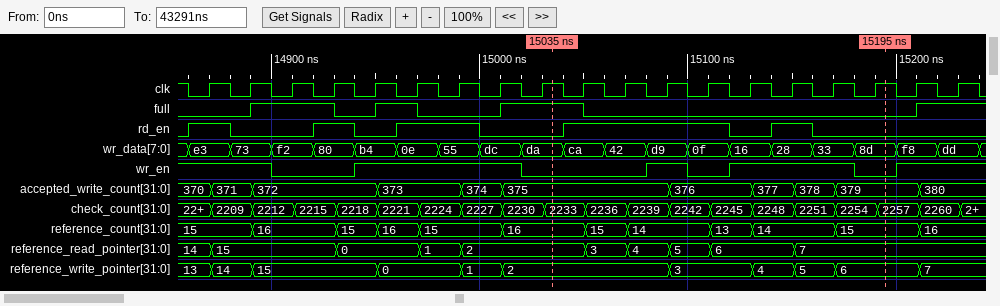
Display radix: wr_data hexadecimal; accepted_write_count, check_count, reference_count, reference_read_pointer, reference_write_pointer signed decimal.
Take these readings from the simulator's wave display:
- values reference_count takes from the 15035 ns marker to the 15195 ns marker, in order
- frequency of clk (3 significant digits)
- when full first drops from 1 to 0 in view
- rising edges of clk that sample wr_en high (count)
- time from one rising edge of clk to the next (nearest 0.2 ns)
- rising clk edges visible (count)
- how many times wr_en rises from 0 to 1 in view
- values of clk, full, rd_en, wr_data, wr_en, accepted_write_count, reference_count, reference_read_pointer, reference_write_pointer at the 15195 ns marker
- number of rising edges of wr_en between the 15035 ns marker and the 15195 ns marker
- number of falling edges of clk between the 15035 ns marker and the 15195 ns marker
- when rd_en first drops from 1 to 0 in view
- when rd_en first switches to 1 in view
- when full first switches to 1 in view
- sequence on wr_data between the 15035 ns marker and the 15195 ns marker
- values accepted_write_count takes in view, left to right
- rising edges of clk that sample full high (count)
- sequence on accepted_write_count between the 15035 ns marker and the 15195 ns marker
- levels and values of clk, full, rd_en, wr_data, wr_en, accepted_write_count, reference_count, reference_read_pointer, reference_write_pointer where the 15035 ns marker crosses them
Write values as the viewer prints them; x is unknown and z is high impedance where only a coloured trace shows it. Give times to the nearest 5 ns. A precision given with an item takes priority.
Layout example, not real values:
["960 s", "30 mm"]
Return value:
["16, 15, 14, 13, 14, 15", "50.0 MHz", "14930 ns", "12", "20 ns", "19", "4", "clk=1, full=0, rd_en=0, wr_data=8d, wr_en=0, accepted_write_count=379, reference_count=15, reference_read_pointer=7, reference_write_pointer=6", "2", "8", "14880 ns", "14860 ns", "14890 ns", "da, ca, 42, d9, 0f, 16, 28, 33, 8d", "370, 371, 372, 373, 374, 375, 376, 377, 378, 379, 380", "6", "375, 376, 377, 378, 379", "clk=1, full=1, rd_en=0, wr_data=da, wr_en=0, accepted_write_count=375, reference_count=16, reference_read_pointer=2, reference_write_pointer=2"]
